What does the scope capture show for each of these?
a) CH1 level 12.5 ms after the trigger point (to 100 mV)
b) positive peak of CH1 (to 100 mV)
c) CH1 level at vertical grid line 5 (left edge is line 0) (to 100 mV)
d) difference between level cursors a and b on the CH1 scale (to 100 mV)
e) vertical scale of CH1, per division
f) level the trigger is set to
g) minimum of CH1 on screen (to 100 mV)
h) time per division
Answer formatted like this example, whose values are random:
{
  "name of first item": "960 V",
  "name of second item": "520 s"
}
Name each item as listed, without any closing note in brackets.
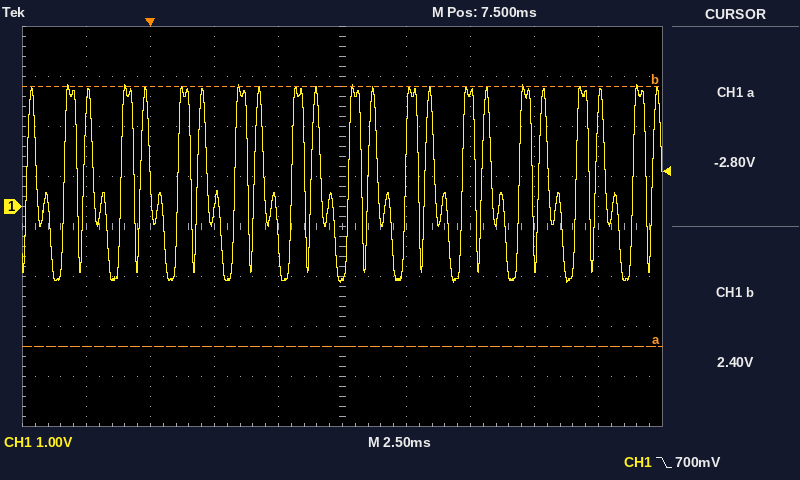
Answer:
{
  "CH1 level 12.5 ms after the trigger point": "2.3 V",
  "positive peak of CH1": "2.4 V",
  "CH1 level at vertical grid line 5 (left edge is line 0)": "-1.4 V",
  "difference between level cursors a and b on the CH1 scale": "5.2 V",
  "vertical scale of CH1, per division": "1 V",
  "level the trigger is set to": "700 mV",
  "minimum of CH1 on screen": "-1.5 V",
  "time per division": "2.5 ms"
}
